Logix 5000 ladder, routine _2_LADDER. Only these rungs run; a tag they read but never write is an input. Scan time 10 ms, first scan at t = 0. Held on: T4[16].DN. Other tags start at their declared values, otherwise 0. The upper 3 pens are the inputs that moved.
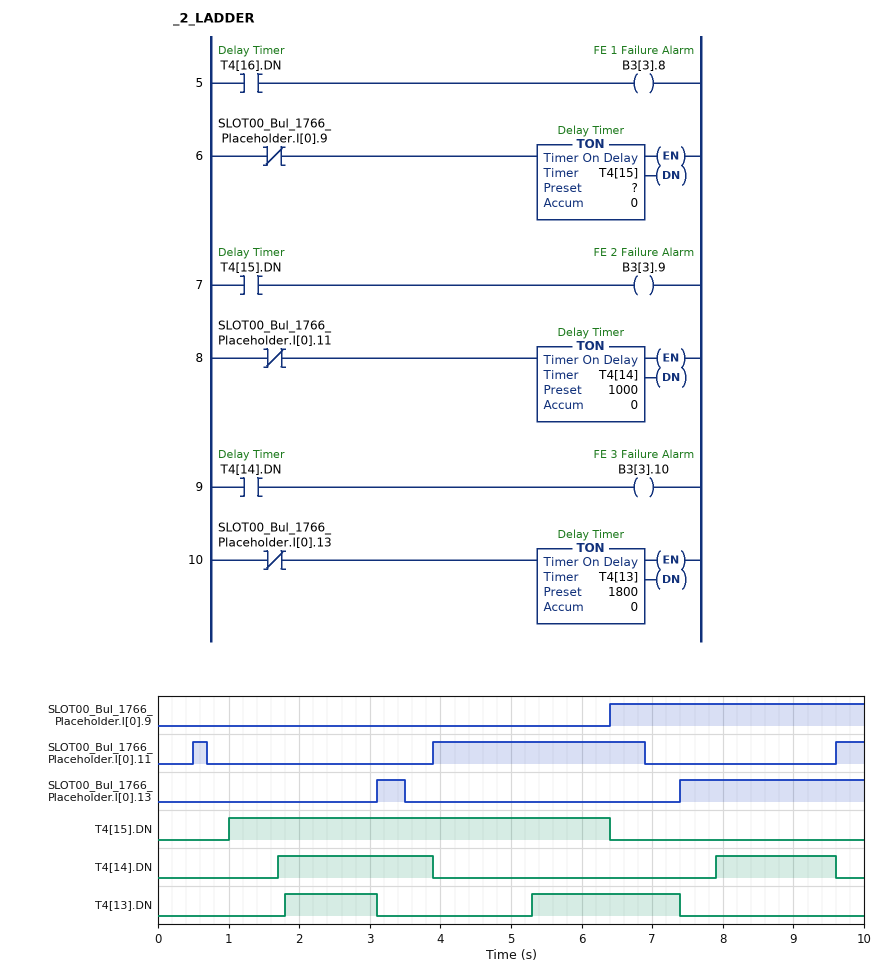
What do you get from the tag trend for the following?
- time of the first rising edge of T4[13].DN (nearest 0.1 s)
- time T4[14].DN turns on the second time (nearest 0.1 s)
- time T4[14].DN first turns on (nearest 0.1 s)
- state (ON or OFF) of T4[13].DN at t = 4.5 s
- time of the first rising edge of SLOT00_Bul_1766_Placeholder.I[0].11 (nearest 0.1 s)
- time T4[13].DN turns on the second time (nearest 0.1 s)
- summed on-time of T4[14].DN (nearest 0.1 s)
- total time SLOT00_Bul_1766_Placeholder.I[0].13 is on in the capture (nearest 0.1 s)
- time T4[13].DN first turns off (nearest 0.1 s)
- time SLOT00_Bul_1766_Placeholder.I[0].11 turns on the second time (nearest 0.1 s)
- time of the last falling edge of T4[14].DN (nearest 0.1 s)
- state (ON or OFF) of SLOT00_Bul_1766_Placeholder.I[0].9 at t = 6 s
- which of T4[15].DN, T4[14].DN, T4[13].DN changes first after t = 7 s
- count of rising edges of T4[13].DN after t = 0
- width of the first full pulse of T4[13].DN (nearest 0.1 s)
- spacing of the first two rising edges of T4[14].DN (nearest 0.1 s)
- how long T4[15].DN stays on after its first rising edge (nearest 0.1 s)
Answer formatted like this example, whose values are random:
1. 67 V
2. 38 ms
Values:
1. 1.8 s
2. 7.9 s
3. 1.7 s
4. OFF
5. 0.5 s
6. 5.3 s
7. 3.9 s
8. 3.0 s
9. 3.1 s
10. 3.9 s
11. 9.6 s
12. OFF
13. T4[13].DN
14. 2
15. 1.3 s
16. 6.2 s
17. 5.4 s
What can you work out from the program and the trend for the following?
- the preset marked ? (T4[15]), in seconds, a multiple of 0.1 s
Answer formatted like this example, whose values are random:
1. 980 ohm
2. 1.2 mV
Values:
1. 1.0 s
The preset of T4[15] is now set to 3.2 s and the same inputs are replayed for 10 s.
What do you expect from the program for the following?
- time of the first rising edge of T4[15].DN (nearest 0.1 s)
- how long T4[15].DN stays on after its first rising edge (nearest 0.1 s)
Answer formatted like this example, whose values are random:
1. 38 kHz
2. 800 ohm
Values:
1. 3.2 s
2. 3.2 s
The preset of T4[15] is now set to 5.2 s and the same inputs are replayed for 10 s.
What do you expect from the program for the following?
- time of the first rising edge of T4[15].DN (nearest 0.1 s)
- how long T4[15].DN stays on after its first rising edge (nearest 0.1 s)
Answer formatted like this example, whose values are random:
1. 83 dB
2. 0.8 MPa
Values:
1. 5.2 s
2. 1.2 s
